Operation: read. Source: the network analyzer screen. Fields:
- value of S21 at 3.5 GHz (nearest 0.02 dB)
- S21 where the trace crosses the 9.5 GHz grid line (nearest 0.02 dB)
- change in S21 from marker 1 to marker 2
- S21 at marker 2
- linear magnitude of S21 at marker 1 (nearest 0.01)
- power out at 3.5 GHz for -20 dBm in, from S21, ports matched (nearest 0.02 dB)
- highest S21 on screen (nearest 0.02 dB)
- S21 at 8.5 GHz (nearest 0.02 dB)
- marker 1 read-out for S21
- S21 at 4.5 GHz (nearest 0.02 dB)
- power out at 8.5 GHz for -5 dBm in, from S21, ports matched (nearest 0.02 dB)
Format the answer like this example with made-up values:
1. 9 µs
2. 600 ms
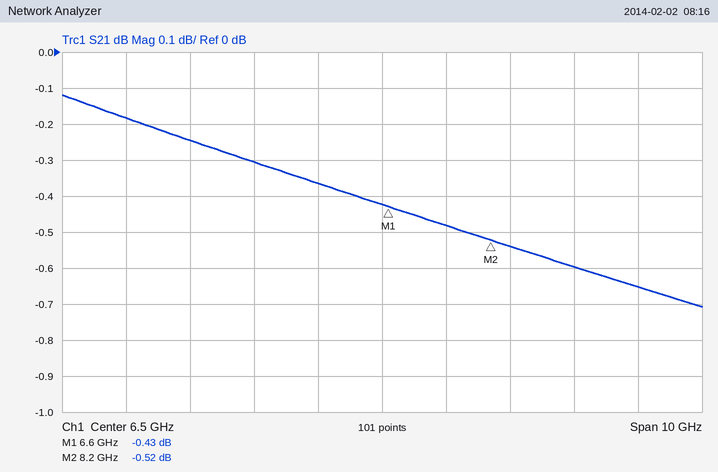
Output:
1. -0.24 dB
2. -0.60 dB
3. -0.09 dB
4. -0.52 dB
5. 0.95
6. -20.24 dBm
7. -0.12 dB
8. -0.54 dB
9. -0.43 dB
10. -0.30 dB
11. -5.54 dBm
